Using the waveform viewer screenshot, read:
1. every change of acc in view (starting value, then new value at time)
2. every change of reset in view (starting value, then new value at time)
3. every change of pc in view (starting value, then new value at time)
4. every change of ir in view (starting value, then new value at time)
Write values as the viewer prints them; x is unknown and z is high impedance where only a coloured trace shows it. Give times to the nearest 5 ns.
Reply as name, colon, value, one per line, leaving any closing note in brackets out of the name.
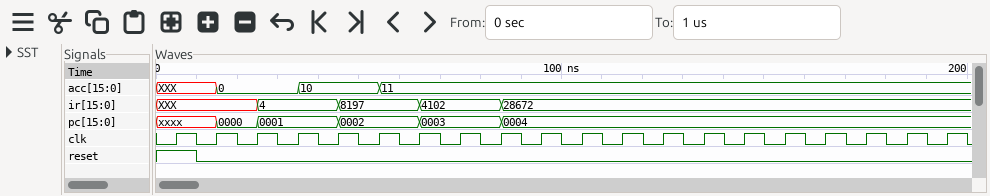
every change of acc in view: XXX, 0 at 15 ns, 10 at 35 ns, 11 at 55 ns
every change of reset in view: 1, 0 at 10 ns
every change of pc in view: xxxx, 0000 at 15 ns, 0001 at 25 ns, 0002 at 45 ns, 0003 at 65 ns, 0004 at 85 ns
every change of ir in view: XXX, 4 at 25 ns, 8197 at 45 ns, 4102 at 65 ns, 28672 at 85 ns
